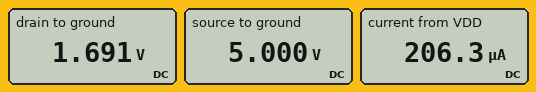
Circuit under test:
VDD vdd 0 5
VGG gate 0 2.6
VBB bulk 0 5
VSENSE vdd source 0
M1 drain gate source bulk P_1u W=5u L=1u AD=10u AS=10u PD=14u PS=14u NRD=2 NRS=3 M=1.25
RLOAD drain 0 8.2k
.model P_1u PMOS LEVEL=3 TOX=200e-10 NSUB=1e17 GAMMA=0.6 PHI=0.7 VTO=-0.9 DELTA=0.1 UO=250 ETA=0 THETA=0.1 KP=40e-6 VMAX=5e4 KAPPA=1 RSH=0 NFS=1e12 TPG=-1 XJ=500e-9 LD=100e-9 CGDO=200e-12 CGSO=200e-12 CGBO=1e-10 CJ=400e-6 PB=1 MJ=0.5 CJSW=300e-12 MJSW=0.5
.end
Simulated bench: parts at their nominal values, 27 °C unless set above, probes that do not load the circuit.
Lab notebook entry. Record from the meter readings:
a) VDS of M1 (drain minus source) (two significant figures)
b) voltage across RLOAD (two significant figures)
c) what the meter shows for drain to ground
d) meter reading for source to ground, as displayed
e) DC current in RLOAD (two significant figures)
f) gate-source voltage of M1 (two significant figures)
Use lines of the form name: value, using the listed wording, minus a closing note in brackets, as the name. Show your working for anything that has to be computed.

VDS of M1 (drain minus source): 1.691 V - 5 V = -3.3 V
voltage across RLOAD: 1.691 V = 1.7 V
what the meter shows for drain to ground: 1.691 V
meter reading for source to ground, as displayed: 5.000 V
DC current in RLOAD: (1.691 V) / 8.2 kΩ = 210 µA
gate-source voltage of M1: 2.6 V - 5 V = -2.4 V
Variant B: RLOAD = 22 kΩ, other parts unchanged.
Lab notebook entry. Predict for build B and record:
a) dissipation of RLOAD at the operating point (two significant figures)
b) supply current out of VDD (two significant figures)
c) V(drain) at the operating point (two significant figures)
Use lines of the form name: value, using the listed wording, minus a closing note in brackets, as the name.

dissipation of RLOAD at the operating point: 680 µW
supply current out of VDD: 180 µA
V(drain) at the operating point: 3.9 V
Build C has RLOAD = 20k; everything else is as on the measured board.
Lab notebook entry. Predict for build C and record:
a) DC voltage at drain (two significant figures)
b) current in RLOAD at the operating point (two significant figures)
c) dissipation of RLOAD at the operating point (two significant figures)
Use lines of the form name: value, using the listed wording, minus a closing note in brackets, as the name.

DC voltage at drain: 3.6 V
current in RLOAD at the operating point: 180 µA
dissipation of RLOAD at the operating point: 660 µW
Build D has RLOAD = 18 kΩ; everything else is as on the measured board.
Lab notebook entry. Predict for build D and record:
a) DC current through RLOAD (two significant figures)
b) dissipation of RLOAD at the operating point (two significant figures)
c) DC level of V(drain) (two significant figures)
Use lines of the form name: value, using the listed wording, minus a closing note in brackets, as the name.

DC current through RLOAD: 190 µA
dissipation of RLOAD at the operating point: 620 µW
DC level of V(drain): 3.3 V
